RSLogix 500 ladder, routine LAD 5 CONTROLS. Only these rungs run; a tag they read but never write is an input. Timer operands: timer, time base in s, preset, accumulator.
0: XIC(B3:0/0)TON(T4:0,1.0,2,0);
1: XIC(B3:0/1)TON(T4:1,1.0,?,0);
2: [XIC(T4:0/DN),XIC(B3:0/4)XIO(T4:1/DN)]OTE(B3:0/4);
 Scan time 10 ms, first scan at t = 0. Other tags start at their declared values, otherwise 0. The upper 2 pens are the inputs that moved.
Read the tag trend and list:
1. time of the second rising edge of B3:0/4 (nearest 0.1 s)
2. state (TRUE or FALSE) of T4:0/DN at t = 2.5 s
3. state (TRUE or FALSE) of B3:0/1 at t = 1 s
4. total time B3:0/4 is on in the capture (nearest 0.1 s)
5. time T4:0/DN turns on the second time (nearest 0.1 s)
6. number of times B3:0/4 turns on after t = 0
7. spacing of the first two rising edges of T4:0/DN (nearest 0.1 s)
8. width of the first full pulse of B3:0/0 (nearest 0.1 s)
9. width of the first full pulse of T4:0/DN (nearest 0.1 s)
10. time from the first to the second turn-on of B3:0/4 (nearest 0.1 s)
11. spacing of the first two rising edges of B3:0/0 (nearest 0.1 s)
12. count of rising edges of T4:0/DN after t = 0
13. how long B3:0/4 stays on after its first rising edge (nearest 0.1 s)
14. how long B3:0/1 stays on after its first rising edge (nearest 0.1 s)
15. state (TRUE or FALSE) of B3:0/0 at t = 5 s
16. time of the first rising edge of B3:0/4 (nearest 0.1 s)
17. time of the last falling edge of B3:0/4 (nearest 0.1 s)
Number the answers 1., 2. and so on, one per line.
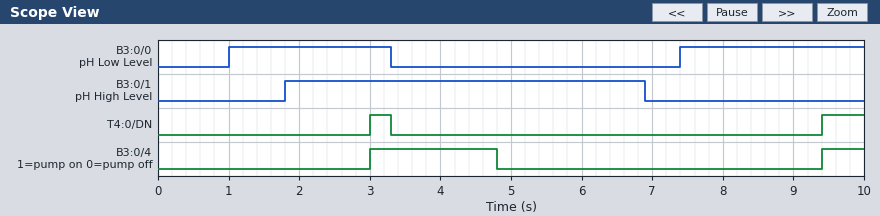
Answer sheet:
1. 9.4 s
2. FALSE
3. FALSE
4. 2.4 s
5. 9.4 s
6. 2
7. 6.4 s
8. 2.3 s
9. 0.3 s
10. 6.4 s
11. 6.4 s
12. 2
13. 1.8 s
14. 5.1 s
15. FALSE
16. 3.0 s
17. 4.8 s
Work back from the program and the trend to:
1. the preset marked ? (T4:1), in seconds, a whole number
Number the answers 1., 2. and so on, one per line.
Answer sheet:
1. 3 s
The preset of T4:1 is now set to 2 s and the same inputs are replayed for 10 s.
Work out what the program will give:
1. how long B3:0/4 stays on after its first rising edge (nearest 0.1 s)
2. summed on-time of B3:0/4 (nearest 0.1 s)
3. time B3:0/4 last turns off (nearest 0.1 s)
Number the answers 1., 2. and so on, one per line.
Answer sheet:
1. 0.8 s
2. 1.4 s
3. 3.8 s
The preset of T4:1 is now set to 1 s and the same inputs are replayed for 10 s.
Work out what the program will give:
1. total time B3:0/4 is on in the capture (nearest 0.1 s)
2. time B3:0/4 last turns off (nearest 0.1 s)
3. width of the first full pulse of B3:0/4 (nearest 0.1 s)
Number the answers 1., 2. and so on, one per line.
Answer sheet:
1. 0.9 s
2. 3.3 s
3. 0.3 s
